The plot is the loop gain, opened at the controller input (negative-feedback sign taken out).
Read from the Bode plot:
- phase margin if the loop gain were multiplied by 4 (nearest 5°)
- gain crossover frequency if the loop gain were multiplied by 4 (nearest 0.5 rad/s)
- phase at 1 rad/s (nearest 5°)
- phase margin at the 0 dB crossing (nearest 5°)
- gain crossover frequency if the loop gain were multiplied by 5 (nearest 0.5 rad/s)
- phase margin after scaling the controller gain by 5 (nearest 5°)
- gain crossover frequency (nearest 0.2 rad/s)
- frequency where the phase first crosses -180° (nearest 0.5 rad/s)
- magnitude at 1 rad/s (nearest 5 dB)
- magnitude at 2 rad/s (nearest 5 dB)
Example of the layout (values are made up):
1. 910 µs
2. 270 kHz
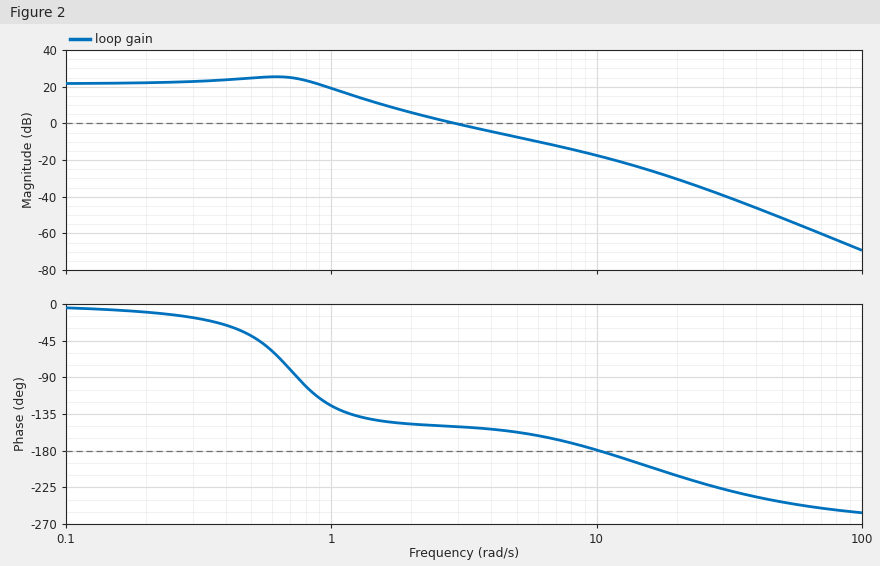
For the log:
1. 15°
2. 7.0 rad/s
3. -125°
4. 30°
5. 8.0 rad/s
6. 10°
7. 3.0 rad/s
8. 10.0 rad/s
9. 20 dB
10. 5 dB
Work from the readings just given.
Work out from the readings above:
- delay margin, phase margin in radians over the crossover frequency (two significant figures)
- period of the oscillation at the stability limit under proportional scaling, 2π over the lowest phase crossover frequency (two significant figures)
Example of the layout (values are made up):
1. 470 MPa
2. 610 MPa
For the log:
1. 0.17 s
2. 0.63 s
